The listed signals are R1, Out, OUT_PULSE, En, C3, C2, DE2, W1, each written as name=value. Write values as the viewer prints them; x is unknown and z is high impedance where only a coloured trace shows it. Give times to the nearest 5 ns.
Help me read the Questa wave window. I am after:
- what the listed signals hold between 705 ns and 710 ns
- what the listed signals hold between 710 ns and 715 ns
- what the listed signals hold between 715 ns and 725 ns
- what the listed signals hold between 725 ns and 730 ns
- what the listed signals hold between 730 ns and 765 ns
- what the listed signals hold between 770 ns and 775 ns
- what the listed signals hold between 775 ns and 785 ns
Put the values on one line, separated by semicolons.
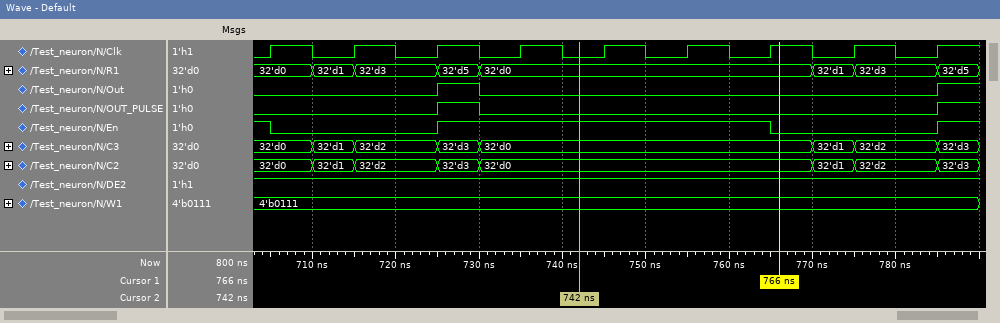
R1=32'd0, Out=0, OUT_PULSE=0, En=0, C3=32'd0, C2=32'd0, DE2=1, W1=4'b0111; R1=32'd1, Out=0, OUT_PULSE=0, En=0, C3=32'd1, C2=32'd1, DE2=1, W1=4'b0111; R1=32'd3, Out=0, OUT_PULSE=0, En=0, C3=32'd2, C2=32'd2, DE2=1, W1=4'b0111; R1=32'd5, Out=1, OUT_PULSE=1, En=1, C3=32'd3, C2=32'd3, DE2=1, W1=4'b0111; R1=32'd0, Out=0, OUT_PULSE=0, En=1, C3=32'd0, C2=32'd0, DE2=1, W1=4'b0111; R1=32'd1, Out=0, OUT_PULSE=0, En=0, C3=32'd1, C2=32'd1, DE2=1, W1=4'b0111; R1=32'd3, Out=0, OUT_PULSE=0, En=0, C3=32'd2, C2=32'd2, DE2=1, W1=4'b0111
